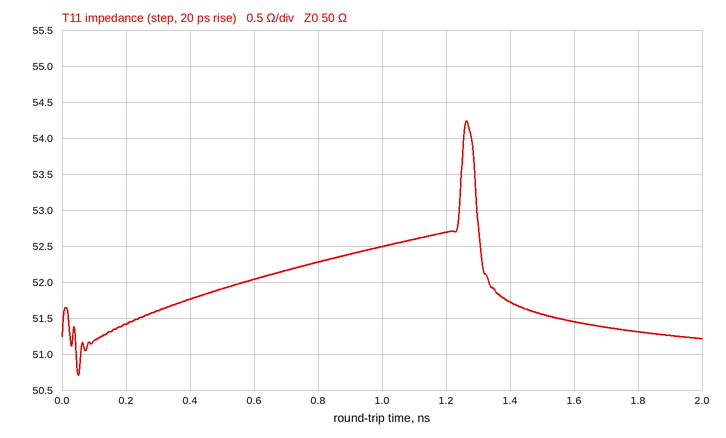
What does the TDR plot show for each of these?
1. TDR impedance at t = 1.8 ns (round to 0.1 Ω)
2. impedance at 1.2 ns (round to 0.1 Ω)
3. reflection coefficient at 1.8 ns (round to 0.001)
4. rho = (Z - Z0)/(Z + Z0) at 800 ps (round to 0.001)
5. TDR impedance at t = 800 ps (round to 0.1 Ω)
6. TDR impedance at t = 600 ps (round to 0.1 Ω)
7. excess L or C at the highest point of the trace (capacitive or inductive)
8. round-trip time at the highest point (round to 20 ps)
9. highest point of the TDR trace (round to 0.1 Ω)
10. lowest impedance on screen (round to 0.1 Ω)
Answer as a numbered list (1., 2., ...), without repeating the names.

1. 51.3 Ω
2. 52.7 Ω
3. +0.013
4. +0.022
5. 52.3 Ω
6. 52.0 Ω
7. inductive
8. 1.26 ns
9. 54.2 Ω
10. 50.7 Ω
